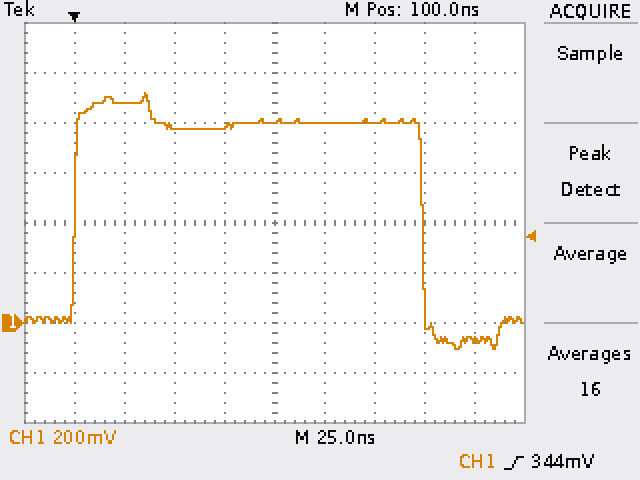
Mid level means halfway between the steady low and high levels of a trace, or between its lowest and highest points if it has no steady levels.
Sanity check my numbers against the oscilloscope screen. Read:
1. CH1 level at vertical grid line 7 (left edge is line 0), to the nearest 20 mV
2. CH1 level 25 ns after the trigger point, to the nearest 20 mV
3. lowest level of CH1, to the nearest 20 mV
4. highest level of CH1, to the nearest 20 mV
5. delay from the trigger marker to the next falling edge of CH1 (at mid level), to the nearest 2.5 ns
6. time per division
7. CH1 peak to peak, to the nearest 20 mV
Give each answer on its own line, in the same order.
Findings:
800 mV
880 mV
-100 mV
920 mV
175.0 ns
25 ns
1.02 V
